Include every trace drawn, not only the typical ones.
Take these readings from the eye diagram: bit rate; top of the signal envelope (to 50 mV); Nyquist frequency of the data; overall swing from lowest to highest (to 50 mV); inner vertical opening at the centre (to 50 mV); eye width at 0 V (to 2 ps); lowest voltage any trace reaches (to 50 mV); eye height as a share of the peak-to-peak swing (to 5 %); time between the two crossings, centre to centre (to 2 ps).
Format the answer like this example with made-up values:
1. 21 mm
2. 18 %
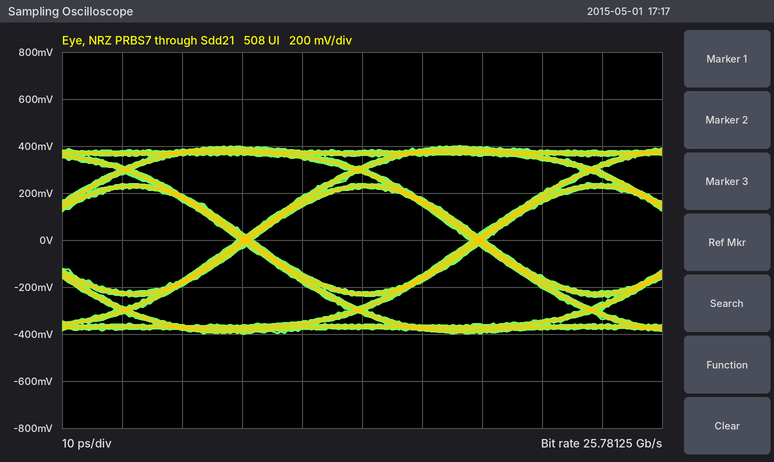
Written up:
1. 25.78125 Gb/s
2. 400 mV
3. 12.89062 GHz
4. 800 mV
5. 450 mV
6. 36 ps
7. -400 mV
8. 55 %
9. 38 ps
